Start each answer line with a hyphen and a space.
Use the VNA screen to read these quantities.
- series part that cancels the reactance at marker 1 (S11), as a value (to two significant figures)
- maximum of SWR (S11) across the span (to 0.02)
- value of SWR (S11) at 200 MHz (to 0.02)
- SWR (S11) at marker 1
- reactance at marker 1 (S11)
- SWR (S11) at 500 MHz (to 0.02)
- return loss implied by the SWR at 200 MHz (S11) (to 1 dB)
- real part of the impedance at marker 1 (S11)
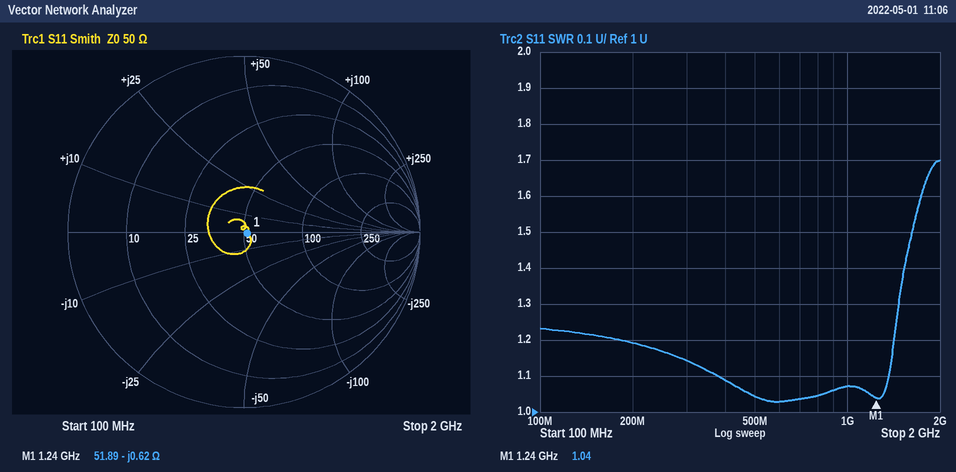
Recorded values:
- 80 pH
- 1.70
- 1.20
- 1.04
- -0.62 Ω
- 1.04
- 21 dB
- 51.89 Ω
